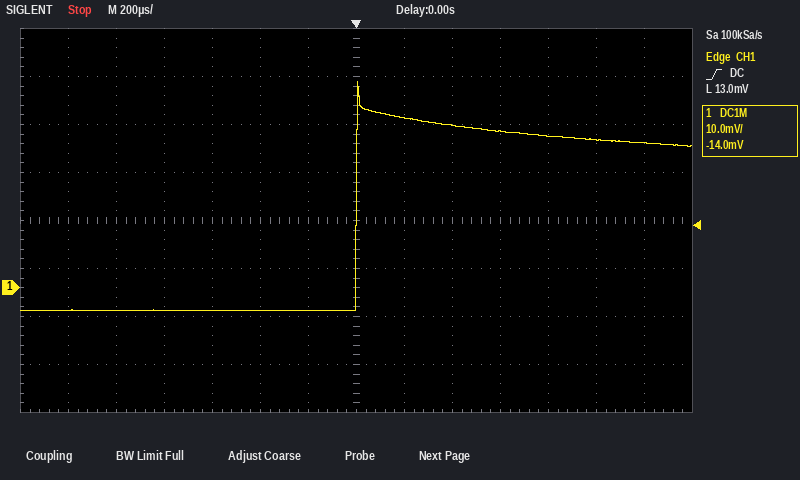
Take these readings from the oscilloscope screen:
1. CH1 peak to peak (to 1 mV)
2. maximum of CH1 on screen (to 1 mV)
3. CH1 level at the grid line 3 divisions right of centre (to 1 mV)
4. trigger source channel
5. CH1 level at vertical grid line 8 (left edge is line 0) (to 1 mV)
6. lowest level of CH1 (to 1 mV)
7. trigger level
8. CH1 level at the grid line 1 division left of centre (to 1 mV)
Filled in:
48 mV
43 mV
33 mV
CH1
35 mV
-5 mV
13.0 mV
-5 mV
